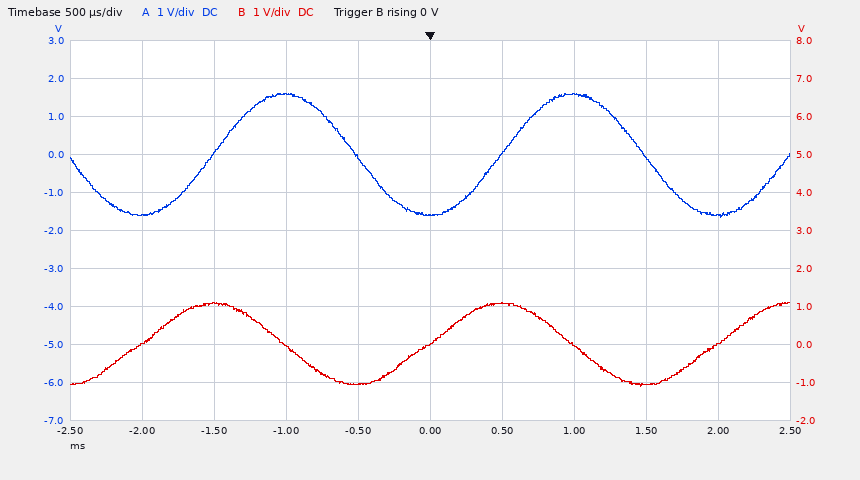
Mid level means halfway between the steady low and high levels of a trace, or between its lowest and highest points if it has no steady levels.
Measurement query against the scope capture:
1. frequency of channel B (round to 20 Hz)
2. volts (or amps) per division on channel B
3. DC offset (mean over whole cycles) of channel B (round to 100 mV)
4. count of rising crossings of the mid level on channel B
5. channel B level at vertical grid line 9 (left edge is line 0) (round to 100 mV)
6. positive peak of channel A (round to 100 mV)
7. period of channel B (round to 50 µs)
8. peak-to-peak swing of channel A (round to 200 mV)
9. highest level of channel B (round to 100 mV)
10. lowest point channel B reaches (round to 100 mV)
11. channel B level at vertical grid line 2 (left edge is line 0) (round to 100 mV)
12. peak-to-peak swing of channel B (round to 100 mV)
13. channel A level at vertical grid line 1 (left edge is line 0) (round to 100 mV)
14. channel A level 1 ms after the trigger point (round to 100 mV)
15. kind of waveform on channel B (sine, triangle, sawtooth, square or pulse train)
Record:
500 Hz
1 V
0.0 V
3
0.0 V
1.6 V
2.00 ms
3.2 V
1.1 V
-1.1 V
1.1 V
2.2 V
-1.6 V
1.6 V
sine
